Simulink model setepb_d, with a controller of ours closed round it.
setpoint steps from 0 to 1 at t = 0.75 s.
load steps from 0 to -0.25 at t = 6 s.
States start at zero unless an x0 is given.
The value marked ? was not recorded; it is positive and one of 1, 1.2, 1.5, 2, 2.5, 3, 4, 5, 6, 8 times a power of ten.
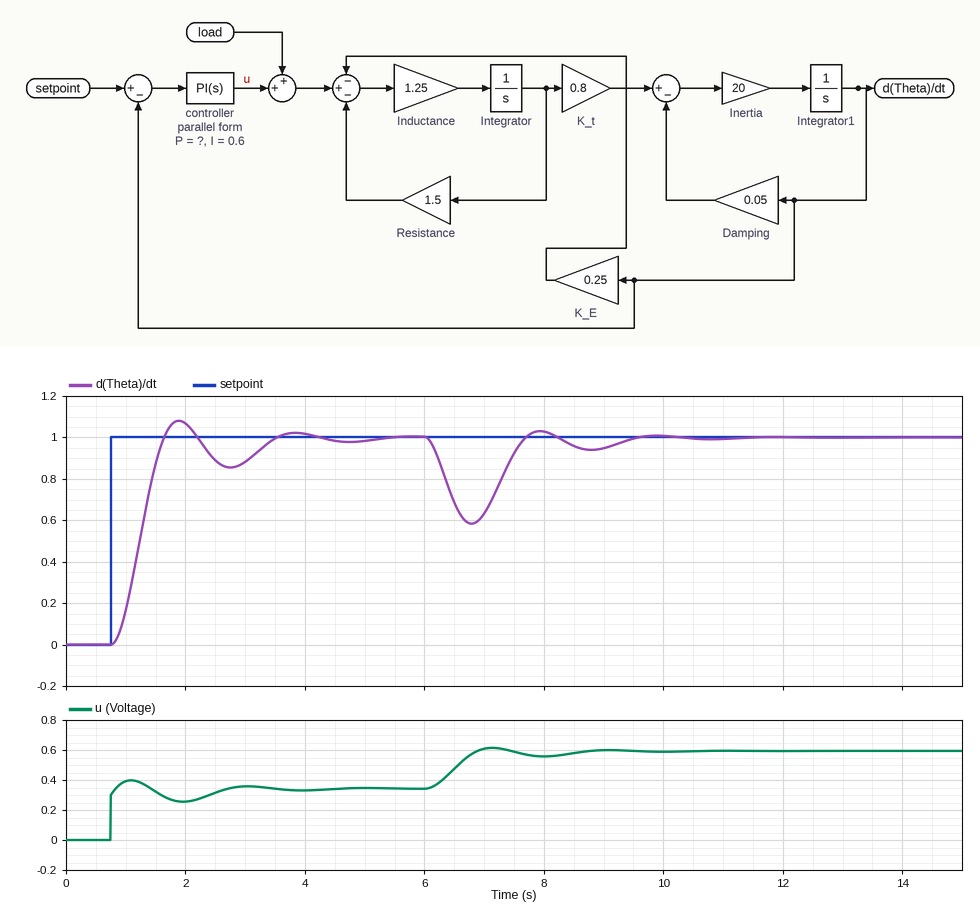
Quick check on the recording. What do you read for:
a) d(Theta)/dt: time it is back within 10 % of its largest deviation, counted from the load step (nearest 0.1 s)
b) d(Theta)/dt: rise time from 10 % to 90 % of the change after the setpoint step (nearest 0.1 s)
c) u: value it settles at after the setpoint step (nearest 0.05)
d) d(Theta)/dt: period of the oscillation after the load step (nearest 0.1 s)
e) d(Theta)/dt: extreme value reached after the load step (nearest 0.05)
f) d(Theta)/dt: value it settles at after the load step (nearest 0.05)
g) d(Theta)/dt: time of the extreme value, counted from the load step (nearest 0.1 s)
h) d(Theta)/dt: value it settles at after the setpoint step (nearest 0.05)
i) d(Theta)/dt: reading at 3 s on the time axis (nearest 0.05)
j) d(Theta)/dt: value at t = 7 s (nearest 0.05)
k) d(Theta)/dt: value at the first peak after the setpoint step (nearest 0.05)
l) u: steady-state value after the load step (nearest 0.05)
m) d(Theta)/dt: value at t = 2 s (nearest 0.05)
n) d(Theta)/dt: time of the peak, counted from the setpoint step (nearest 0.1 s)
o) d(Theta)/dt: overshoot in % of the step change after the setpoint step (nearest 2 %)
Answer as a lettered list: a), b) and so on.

a) 3.1 s
b) 0.6 s
c) 0.35
d) 2.0 s
e) 0.60
f) 1.00
g) 0.8 s
h) 1.00
i) 0.90
j) 0.65
k) 1.10
l) 0.60
m) 1.05
n) 1.1 s
o) 8 %
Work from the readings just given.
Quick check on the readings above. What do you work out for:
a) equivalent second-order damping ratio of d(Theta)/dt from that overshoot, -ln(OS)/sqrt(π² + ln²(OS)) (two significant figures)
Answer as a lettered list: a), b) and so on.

a) 0.63
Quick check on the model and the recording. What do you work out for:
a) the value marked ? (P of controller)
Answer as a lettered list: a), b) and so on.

a) 0.3
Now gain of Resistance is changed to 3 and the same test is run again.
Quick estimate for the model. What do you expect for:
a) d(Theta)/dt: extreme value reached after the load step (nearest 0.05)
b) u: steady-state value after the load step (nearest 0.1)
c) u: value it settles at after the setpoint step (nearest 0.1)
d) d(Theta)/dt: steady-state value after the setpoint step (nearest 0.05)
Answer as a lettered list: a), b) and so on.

a) 0.70
b) 0.7
c) 0.4
d) 1.00
